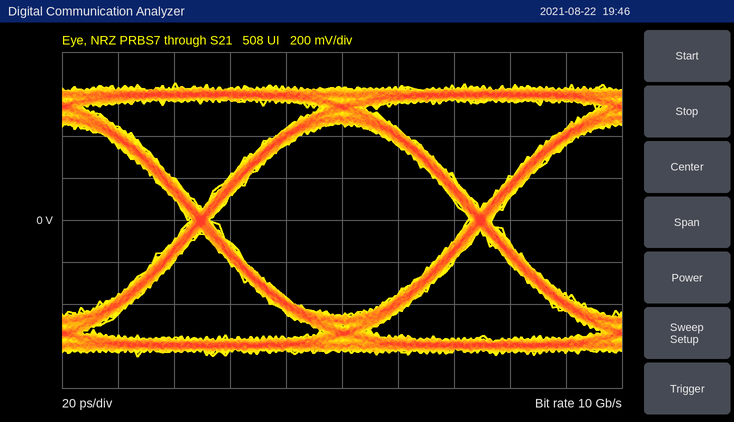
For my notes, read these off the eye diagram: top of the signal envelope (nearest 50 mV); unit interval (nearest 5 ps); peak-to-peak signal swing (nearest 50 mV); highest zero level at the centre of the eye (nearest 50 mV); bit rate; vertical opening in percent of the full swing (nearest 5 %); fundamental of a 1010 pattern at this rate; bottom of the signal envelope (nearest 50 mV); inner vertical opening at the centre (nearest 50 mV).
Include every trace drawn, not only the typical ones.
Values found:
650 mV
100 ps
1.30 V
-450 mV
10 Gb/s
70 %
5 GHz
-650 mV
900 mV
